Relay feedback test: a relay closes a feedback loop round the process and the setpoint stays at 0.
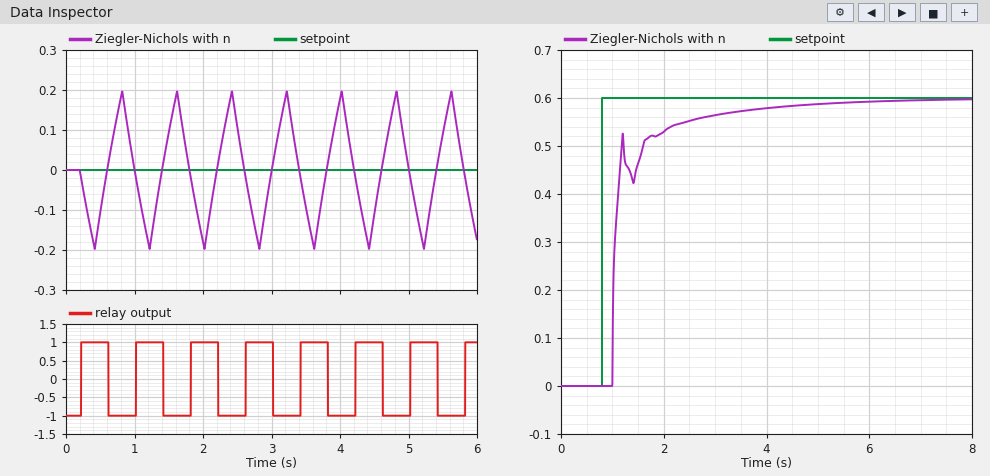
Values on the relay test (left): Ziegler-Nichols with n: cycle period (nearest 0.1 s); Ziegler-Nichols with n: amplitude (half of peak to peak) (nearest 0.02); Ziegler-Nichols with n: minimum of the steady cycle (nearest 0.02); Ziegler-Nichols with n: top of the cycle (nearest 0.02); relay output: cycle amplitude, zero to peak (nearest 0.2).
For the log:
0.8 s
0.20
-0.20
0.20
1.0
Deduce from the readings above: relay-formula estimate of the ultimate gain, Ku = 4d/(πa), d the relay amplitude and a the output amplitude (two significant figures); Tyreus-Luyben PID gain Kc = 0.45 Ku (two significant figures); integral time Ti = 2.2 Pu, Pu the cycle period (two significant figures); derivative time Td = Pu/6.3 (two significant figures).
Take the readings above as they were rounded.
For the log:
6.4
2.9
1.8 s
0.13 s
